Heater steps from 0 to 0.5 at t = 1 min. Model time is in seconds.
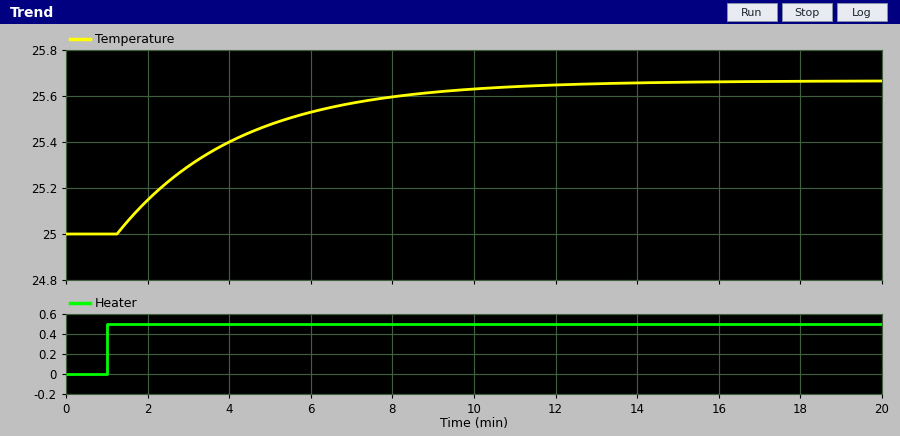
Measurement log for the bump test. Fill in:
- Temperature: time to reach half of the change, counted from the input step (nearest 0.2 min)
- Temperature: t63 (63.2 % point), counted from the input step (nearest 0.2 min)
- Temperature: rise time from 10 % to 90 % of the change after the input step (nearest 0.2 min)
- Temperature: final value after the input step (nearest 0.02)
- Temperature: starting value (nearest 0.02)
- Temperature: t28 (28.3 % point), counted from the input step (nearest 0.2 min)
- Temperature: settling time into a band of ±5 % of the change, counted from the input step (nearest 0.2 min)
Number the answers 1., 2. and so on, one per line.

1. 2.4 min
2. 3.2 min
3. 6.6 min
4. 25.66
5. 25.00
6. 1.2 min
7. 9.2 min
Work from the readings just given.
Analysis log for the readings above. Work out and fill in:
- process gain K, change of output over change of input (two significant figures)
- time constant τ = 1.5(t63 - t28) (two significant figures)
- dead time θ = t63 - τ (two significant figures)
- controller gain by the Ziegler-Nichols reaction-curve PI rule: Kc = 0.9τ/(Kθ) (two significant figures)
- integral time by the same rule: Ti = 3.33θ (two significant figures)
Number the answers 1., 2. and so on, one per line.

1. 1.3
2. 3.0 min
3. 0.20 min
4. 10
5. 0.67 min
